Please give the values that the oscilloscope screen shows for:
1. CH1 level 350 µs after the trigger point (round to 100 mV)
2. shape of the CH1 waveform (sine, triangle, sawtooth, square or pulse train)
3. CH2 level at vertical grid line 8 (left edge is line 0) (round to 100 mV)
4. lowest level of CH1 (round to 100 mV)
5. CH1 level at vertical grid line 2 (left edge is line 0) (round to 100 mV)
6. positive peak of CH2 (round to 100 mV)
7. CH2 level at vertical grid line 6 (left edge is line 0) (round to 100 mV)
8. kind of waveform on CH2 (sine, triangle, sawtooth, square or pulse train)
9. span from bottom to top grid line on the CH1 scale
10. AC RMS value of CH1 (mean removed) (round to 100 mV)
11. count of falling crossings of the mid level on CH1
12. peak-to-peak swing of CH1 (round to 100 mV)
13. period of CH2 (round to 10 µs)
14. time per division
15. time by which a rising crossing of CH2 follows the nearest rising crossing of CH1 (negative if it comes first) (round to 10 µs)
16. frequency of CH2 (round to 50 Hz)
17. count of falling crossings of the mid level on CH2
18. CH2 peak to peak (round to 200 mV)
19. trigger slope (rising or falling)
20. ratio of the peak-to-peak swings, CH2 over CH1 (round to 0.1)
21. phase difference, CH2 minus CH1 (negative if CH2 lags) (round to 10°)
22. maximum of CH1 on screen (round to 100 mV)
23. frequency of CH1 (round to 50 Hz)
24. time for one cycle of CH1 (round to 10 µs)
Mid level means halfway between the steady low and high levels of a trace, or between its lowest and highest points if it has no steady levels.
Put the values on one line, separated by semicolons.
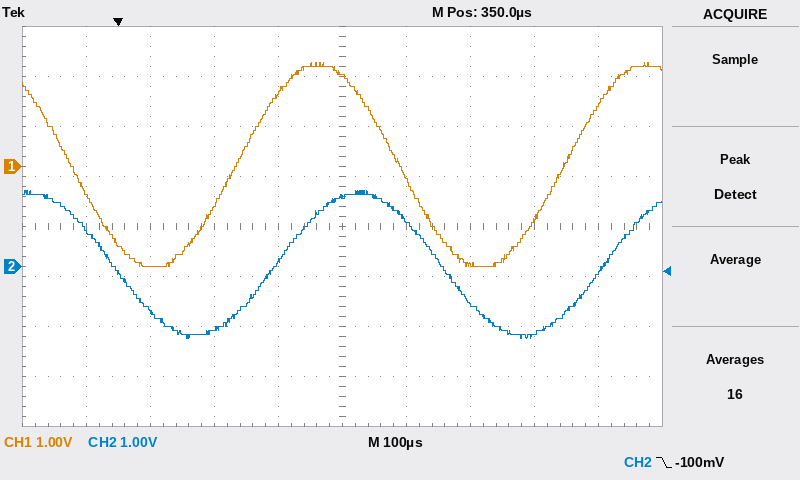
1.8 V; sine; -1.3 V; -2.0 V; -2.0 V; 1.5 V; 900 mV; sine; 8 V; 1.4 V; 2; 4.1 V; 510 µs; 100 µs; +60 µs; 1.95 kHz; 2; 3.0 V; falling; 0.7; -40°; 2.1 V; 1.95 kHz; 510 µs
